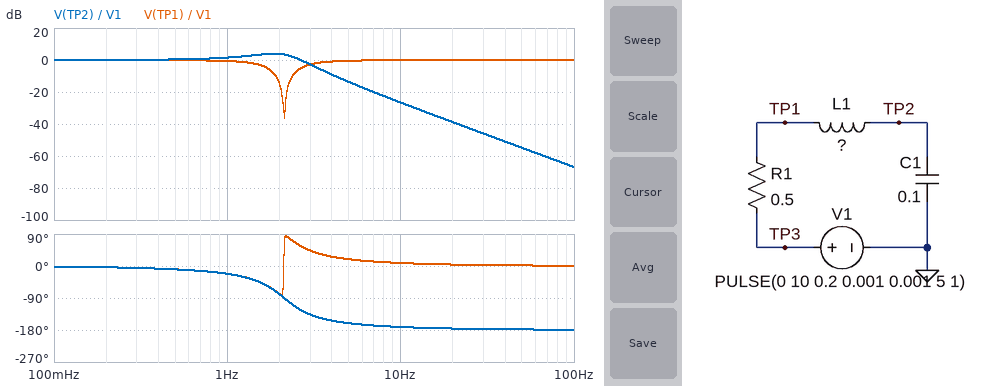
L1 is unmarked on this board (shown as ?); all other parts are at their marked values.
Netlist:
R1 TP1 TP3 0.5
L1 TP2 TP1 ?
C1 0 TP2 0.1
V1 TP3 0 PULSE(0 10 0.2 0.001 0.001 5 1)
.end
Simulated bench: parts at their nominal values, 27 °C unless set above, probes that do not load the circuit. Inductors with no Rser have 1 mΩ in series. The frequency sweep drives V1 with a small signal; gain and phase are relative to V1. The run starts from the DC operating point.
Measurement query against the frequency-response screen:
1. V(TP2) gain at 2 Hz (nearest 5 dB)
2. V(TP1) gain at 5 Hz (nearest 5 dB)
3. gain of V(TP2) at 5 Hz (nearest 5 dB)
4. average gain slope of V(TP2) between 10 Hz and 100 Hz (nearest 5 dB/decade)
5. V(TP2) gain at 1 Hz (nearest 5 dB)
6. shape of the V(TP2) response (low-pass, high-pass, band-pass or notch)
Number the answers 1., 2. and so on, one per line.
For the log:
1. 5 dB
2. 0 dB
3. -15 dB
4. -40 dB/decade
5. 0 dB
6. low-pass
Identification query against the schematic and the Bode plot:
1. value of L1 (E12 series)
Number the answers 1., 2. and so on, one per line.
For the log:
1. 56 mH
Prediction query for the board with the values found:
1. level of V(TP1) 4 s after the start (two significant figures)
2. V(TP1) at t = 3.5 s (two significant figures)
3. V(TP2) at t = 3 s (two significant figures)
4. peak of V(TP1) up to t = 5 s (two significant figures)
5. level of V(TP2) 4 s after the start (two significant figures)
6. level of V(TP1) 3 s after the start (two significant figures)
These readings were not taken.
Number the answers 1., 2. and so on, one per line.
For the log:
1. 10 V
2. 10 V
3. 10 V
4. 11 V
5. 10 V
6. 10 V
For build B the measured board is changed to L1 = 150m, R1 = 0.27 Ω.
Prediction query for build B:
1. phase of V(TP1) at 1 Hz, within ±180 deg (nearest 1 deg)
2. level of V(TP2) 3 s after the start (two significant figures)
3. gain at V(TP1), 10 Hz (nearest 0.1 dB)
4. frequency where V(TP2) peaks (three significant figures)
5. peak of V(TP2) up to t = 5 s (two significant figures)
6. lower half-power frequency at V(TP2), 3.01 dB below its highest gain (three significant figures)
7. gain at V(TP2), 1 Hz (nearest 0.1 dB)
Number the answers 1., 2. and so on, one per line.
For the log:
1. -23 deg
2. 11 V
3. 0 dB
4. 1.28 Hz
5. 17 V
6. 1.13 Hz
7. 7.1 dB
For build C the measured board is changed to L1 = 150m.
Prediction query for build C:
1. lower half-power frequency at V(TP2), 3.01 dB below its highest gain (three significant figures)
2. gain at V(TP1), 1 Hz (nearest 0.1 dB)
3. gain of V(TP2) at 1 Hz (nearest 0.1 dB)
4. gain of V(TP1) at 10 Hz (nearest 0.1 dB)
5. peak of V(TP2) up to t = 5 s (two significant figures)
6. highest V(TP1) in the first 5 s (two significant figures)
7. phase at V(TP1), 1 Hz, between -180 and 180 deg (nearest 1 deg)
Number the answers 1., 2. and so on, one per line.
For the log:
1. 933 mHz
2. -2.0 dB
3. 5.8 dB
4. 0 dB
5. 15 V
6. 12 V
7. -38 deg
